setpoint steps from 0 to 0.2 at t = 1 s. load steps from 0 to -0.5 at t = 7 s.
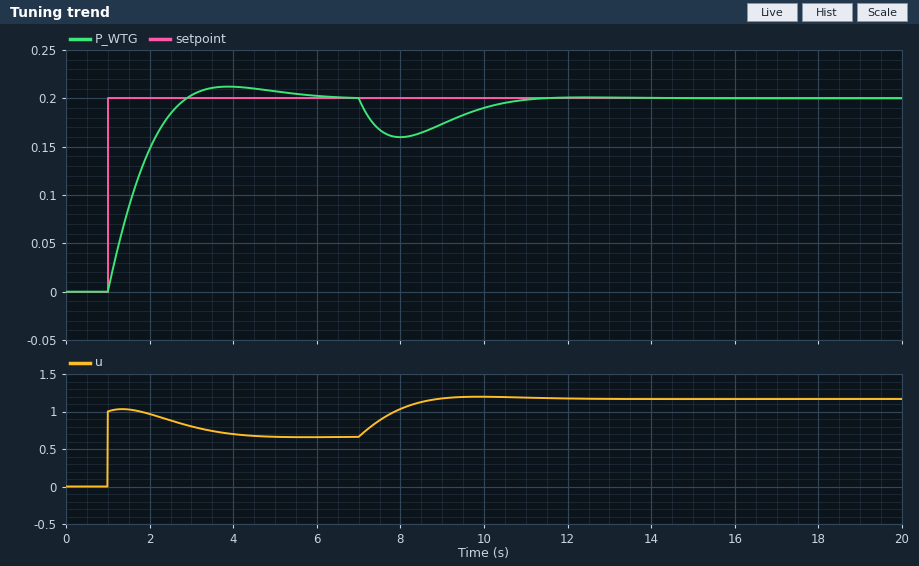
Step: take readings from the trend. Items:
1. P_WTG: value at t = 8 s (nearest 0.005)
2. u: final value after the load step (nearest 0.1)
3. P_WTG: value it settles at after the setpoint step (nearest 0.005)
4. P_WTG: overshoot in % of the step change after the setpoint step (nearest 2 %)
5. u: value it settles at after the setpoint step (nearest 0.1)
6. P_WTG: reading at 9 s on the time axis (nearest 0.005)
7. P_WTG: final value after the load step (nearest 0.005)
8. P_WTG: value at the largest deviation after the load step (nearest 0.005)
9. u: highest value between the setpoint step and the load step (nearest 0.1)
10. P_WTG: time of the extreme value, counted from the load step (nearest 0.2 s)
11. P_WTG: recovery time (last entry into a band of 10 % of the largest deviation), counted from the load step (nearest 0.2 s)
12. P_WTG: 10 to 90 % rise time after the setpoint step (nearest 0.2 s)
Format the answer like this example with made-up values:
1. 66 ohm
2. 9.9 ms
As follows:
1. 0.160
2. 1.2
3. 0.200
4. 6 %
5. 0.7
6. 0.175
7. 0.200
8. 0.160
9. 1.0
10. 1.0 s
11. 3.6 s
12. 1.4 s
